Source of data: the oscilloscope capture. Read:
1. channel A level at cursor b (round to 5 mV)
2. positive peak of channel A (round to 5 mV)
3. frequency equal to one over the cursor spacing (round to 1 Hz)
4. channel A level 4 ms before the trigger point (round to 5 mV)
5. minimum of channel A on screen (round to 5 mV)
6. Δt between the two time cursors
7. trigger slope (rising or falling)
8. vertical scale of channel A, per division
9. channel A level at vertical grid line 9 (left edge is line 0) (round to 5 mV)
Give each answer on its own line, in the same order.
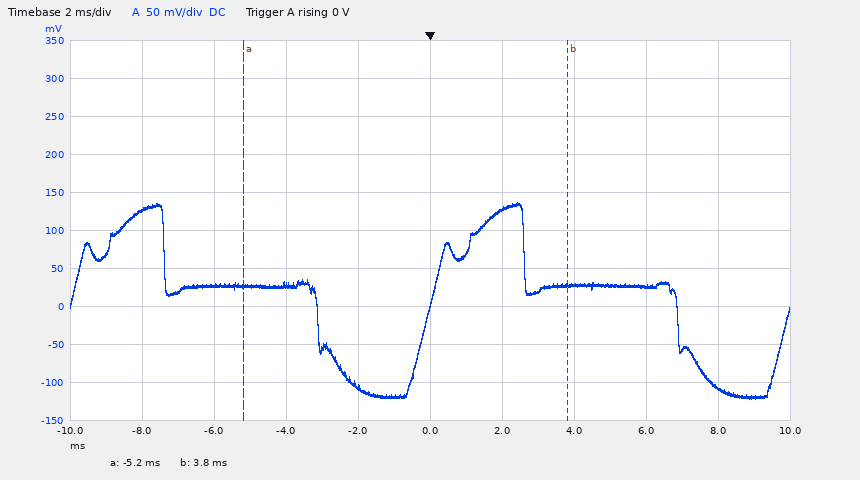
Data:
30 mV
135 mV
111 Hz
30 mV
-120 mV
9.0 ms
rising
50 mV
-105 mV
